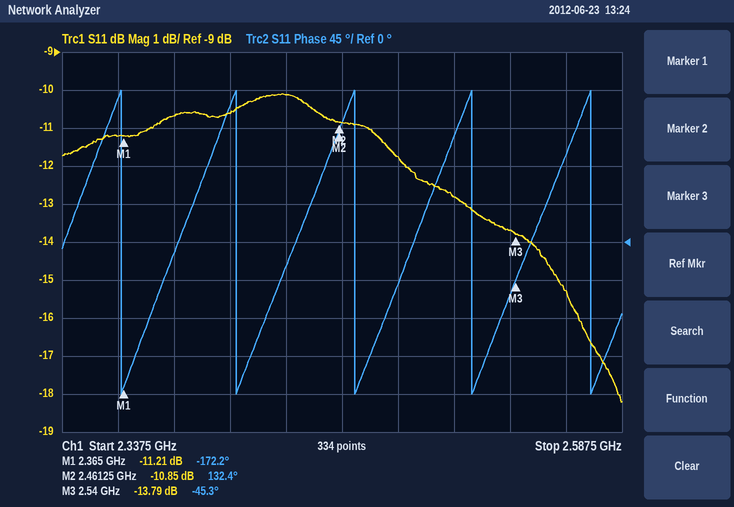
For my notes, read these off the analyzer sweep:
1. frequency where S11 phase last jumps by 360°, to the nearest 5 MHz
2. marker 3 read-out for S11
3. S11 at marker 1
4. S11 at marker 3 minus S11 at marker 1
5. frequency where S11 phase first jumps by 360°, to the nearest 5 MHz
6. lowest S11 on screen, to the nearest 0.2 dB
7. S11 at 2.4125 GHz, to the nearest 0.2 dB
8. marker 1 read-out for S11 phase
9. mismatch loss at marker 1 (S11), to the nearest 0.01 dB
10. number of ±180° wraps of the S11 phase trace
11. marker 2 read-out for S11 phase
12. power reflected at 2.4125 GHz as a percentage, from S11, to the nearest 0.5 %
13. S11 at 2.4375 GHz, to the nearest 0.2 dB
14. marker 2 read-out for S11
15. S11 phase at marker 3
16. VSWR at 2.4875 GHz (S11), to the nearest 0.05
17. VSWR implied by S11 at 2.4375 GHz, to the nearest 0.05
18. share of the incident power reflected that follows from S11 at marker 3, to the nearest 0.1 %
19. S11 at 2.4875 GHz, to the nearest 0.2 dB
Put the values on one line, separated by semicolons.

2.575 GHz; -13.79 dB; -11.21 dB; -2.58 dB; 2.365 GHz; -18.2 dB; -10.6 dB; -172.2°; 0.34 dB; 5; 132.4°; 8.5 %; -10.2 dB; -10.85 dB; -45.3°; 1.70; 1.90; 4.2 %; -11.8 dB
